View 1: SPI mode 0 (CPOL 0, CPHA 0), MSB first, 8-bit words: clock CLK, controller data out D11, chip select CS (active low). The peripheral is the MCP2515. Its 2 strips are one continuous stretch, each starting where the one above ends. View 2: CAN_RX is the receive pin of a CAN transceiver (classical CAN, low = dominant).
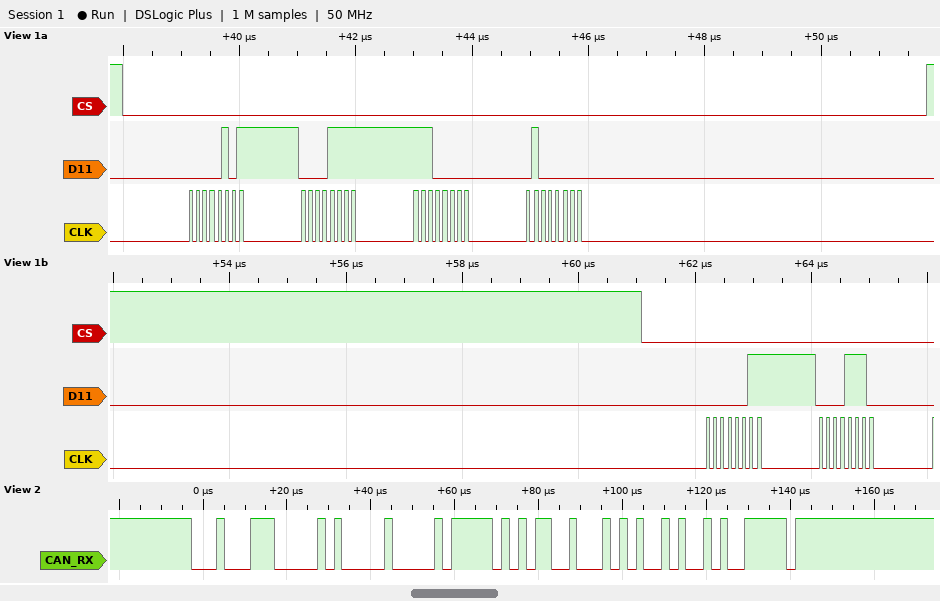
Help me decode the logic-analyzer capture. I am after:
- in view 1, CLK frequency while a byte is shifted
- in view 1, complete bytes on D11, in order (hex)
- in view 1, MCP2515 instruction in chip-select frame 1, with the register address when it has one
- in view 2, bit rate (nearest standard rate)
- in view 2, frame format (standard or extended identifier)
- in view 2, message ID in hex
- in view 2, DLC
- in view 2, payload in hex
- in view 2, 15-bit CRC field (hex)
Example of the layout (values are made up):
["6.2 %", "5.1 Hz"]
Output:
["8 MHz", "05 0F E0 40 03 0E", "BIT MODIFY 0x0F", "500 kbit/s", "standard", "0x11C", "4", "00 7E B2 2A", "0x294F"]
